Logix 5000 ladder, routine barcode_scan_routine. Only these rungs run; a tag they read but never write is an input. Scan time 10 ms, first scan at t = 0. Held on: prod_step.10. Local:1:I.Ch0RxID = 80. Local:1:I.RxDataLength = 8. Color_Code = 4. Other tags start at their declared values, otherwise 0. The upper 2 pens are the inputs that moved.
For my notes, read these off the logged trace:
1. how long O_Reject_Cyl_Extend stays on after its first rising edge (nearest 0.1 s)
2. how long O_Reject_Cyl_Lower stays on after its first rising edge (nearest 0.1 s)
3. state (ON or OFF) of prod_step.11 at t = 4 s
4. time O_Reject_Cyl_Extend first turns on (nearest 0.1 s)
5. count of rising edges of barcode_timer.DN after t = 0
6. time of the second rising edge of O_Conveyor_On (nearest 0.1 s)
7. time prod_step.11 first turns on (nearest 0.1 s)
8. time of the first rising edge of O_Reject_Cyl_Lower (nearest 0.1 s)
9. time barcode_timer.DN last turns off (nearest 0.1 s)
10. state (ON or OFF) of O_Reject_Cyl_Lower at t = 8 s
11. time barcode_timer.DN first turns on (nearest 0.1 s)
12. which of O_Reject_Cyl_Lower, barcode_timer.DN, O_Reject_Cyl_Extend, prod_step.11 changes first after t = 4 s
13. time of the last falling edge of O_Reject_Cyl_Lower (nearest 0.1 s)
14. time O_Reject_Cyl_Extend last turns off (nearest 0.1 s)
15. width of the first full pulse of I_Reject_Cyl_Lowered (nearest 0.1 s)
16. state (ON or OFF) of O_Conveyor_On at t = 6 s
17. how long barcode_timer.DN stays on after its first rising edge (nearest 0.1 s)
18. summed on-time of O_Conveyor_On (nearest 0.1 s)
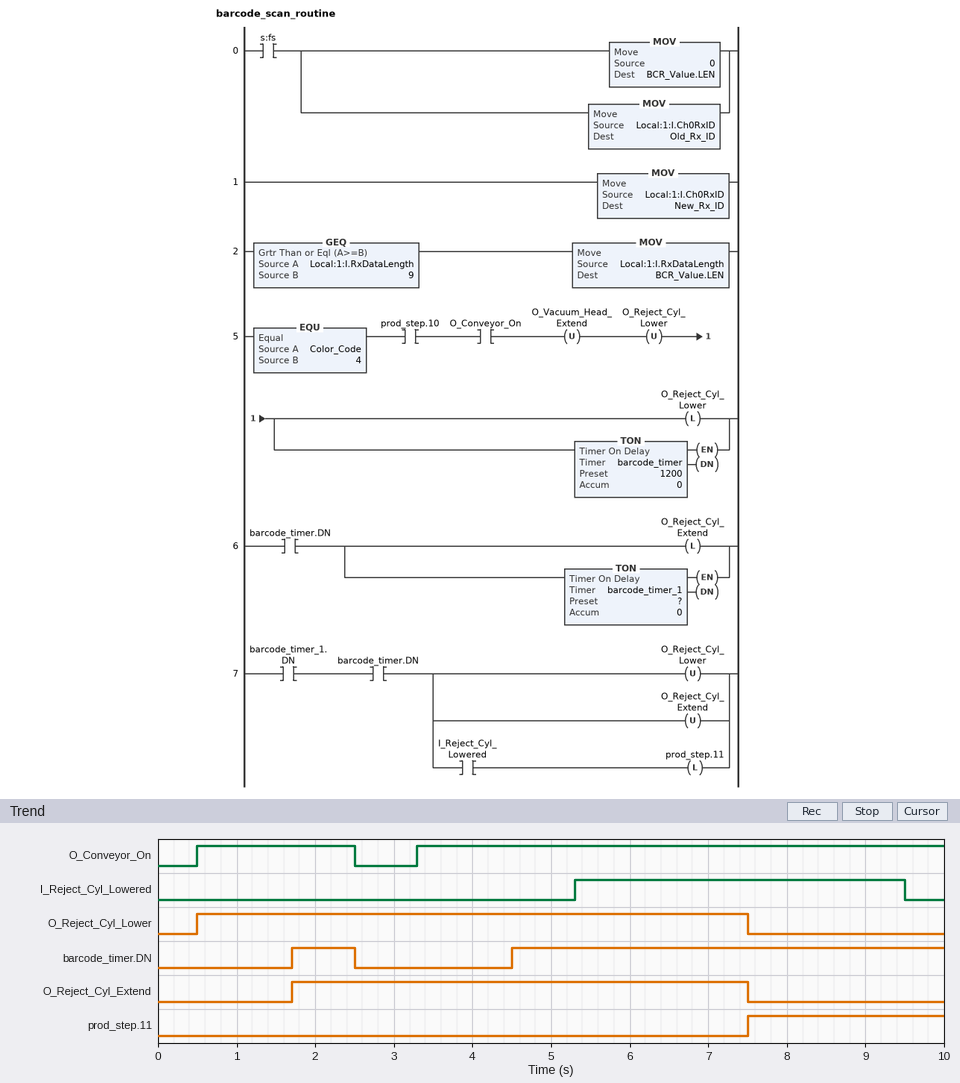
5.8 s
7.0 s
OFF
1.7 s
2
3.3 s
7.5 s
0.5 s
2.5 s
OFF
1.7 s
barcode_timer.DN
7.5 s
7.5 s
4.2 s
ON
0.8 s
8.7 s
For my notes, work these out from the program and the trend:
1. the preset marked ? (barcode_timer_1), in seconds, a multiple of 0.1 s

3.0 s
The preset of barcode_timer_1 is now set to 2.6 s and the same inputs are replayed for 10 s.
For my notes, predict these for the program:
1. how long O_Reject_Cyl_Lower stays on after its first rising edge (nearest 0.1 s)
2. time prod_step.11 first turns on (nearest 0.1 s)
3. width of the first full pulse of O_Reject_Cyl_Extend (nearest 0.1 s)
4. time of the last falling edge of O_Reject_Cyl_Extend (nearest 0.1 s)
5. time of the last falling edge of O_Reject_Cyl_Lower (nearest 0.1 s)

6.6 s
7.1 s
5.4 s
7.1 s
7.1 s
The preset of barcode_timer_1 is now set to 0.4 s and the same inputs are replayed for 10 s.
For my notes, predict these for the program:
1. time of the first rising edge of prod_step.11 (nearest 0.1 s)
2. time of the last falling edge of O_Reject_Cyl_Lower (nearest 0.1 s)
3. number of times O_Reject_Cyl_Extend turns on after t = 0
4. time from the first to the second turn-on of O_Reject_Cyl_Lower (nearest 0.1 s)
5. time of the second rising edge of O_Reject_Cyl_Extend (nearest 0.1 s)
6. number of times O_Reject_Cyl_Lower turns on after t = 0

5.3 s
4.9 s
2
2.8 s
4.5 s
2
